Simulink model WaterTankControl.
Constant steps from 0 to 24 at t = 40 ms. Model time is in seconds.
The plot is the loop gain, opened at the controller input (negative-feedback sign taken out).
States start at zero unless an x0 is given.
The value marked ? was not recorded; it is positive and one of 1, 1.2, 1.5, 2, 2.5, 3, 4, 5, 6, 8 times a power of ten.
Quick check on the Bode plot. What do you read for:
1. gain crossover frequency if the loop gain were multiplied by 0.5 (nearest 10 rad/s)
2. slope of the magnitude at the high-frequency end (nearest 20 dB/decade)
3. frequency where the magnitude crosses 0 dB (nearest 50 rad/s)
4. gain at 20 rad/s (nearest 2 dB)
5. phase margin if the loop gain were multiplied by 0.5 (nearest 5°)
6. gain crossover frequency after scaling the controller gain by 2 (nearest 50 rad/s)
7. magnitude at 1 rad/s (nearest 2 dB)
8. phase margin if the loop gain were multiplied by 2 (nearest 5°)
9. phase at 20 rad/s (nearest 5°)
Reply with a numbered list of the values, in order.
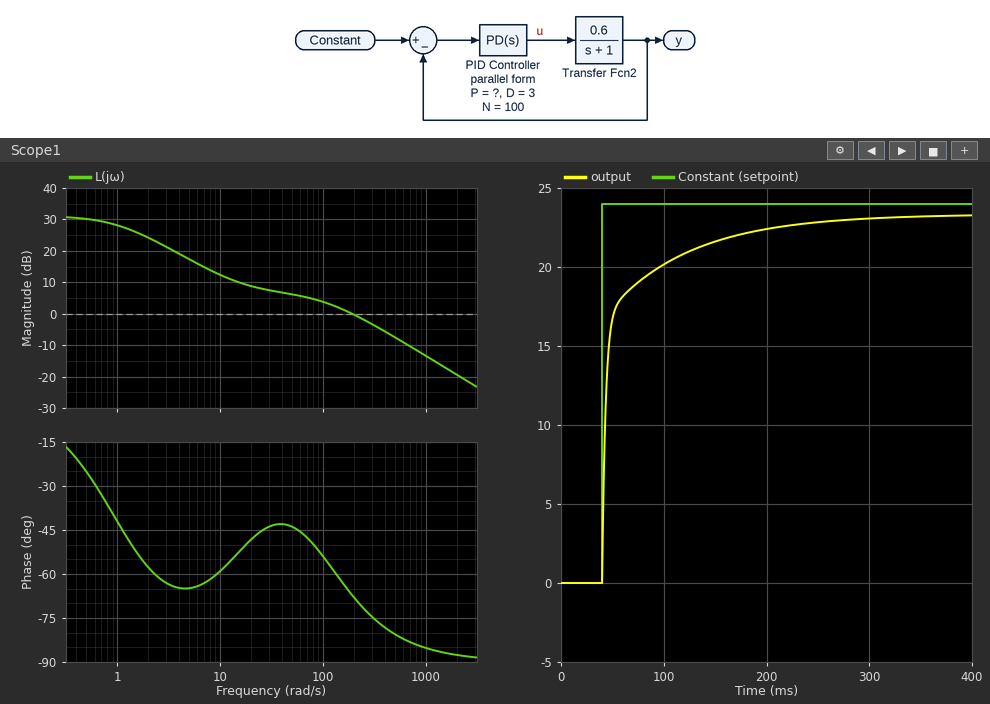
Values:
1. 50 rad/s
2. -20 dB/decade
3. 200 rad/s
4. 8 dB
5. 135°
6. 400 rad/s
7. 28 dB
8. 100°
9. -50°
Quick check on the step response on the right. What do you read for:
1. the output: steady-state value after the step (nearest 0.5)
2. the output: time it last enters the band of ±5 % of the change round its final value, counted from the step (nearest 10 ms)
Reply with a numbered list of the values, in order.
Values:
1. 23.5
2. 140 ms
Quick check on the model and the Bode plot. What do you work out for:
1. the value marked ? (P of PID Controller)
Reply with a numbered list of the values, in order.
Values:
1. 60
